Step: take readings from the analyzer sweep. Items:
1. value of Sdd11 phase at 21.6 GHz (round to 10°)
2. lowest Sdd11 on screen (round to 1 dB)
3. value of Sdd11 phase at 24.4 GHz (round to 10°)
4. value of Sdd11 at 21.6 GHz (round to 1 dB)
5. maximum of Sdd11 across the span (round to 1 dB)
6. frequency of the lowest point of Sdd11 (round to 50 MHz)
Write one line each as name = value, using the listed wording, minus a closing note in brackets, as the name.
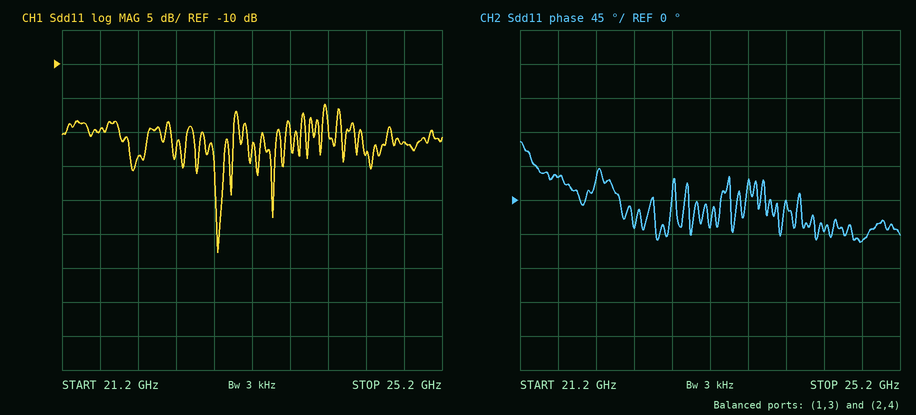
value of Sdd11 phase at 21.6 GHz = 30°
lowest Sdd11 on screen = -38 dB
value of Sdd11 phase at 24.4 GHz = -40°
value of Sdd11 at 21.6 GHz = -20 dB
maximum of Sdd11 across the span = -16 dB
frequency of the lowest point of Sdd11 = 22.85 GHz
